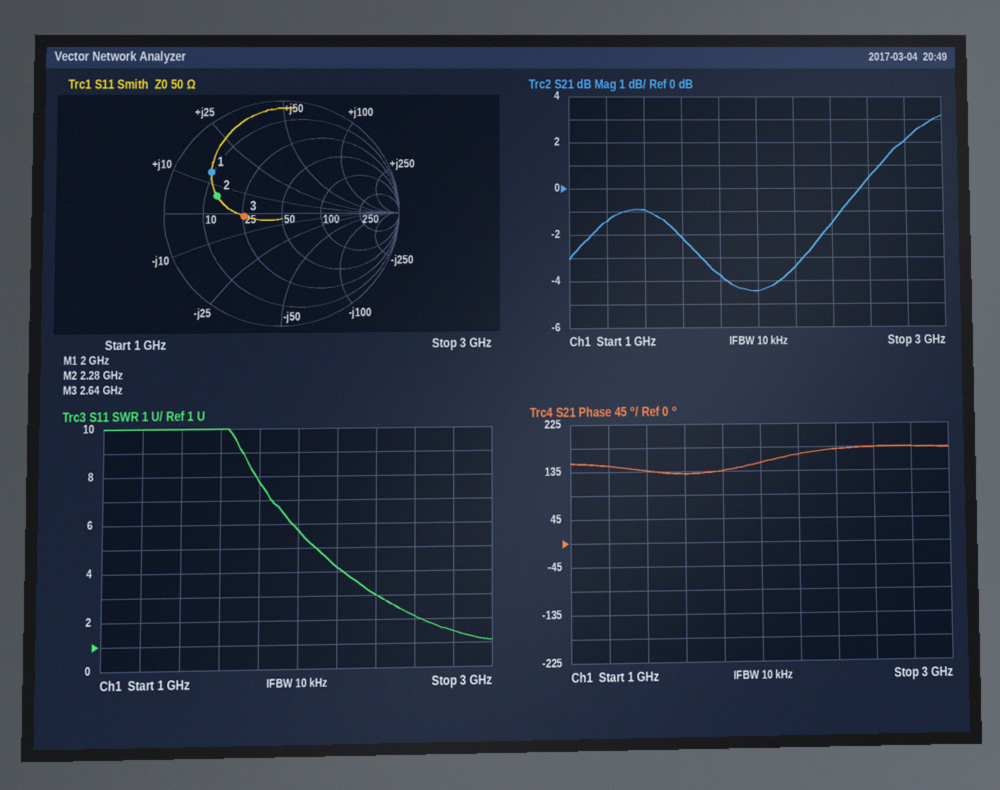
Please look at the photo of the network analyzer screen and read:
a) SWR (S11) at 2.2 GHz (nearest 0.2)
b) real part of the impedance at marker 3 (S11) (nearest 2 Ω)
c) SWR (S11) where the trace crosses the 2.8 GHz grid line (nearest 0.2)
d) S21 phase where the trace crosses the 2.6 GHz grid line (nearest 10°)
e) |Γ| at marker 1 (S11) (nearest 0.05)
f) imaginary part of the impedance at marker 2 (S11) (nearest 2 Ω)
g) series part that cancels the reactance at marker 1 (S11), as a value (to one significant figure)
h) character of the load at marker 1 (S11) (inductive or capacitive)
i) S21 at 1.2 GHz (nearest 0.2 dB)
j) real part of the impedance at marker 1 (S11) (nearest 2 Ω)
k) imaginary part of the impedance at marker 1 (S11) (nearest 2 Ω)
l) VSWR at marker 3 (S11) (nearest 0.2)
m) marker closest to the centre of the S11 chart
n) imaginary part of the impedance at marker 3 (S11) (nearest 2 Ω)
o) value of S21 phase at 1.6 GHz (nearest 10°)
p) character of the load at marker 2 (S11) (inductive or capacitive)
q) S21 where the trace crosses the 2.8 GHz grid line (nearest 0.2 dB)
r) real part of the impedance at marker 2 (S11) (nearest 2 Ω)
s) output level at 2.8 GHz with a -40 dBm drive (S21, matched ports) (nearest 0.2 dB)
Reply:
4.2
26 Ω
1.4
180°
0.70
+6 Ω
6 pF
inductive
-1.4 dB
10 Ω
+14 Ω
2.0
marker 3
-2 Ω
130°
inductive
2.0 dB
14 Ω
-38.0 dBm
